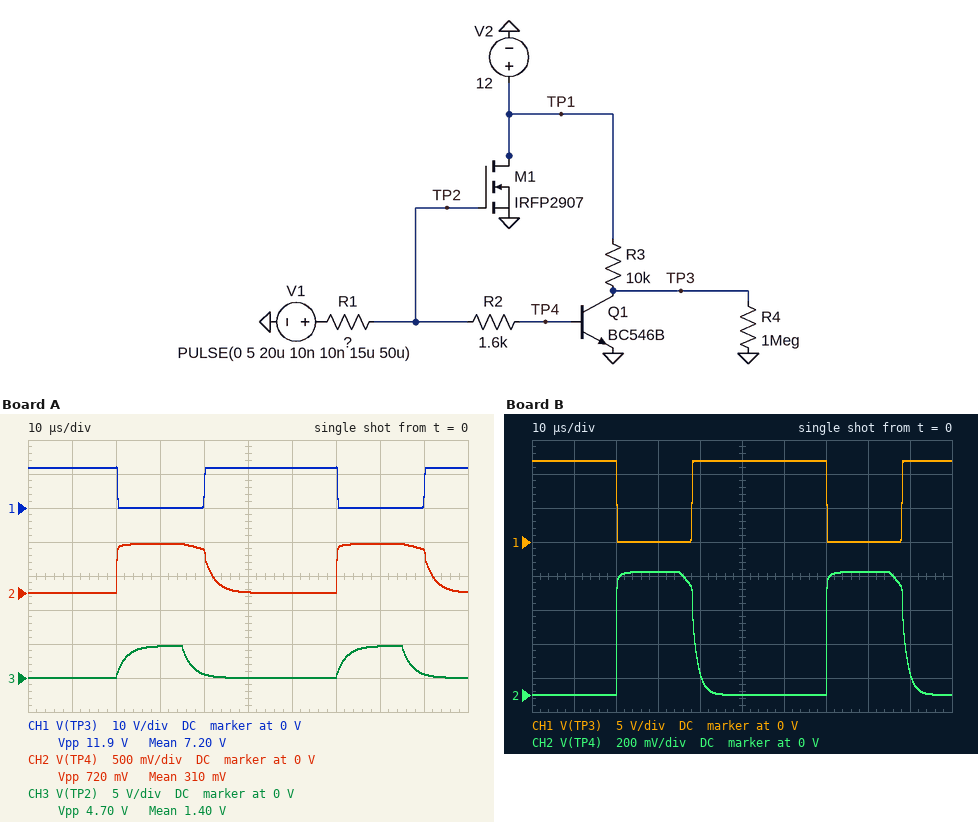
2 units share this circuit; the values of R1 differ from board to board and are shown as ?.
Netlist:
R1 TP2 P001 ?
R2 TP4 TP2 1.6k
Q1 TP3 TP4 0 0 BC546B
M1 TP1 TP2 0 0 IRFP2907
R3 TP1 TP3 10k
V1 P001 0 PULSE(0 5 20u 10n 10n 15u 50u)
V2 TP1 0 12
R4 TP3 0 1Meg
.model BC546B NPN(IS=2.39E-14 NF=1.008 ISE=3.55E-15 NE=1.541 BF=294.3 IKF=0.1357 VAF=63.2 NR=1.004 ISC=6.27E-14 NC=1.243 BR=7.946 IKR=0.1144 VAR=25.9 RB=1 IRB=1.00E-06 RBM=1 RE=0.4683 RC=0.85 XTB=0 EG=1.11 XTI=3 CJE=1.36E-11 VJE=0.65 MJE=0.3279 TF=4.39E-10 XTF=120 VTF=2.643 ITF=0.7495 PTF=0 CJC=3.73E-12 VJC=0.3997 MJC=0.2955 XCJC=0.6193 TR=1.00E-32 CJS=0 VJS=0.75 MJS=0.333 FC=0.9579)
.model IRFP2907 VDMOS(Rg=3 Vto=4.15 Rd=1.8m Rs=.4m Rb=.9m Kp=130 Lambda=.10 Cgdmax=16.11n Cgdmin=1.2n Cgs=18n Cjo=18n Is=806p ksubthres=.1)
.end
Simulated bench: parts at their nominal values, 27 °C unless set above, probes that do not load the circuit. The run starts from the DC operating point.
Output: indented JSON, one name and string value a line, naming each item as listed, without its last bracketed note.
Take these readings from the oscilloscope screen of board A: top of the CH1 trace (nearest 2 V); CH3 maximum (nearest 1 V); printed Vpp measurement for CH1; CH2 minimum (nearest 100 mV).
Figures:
{
  "top of the CH1 trace": "12 V",
  "CH3 maximum": "5 V",
  "printed Vpp measurement for CH1": "11.9 V",
  "CH2 minimum": "0 V"
}
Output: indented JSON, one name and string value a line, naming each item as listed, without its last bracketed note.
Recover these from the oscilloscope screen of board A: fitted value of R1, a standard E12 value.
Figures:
{
  "fitted value of R1, a standard E12 value": "120 Ω"
}
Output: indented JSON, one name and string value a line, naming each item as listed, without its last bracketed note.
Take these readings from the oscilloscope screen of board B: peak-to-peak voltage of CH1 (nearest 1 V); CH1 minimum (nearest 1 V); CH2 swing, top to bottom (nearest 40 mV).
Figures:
{
  "peak-to-peak voltage of CH1": "12 V",
  "CH1 minimum": "0 V",
  "CH2 swing, top to bottom": "720 mV"
}
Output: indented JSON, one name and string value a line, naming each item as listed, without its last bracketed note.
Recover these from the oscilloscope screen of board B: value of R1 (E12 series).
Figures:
{
  "value of R1": "68 Ω"
}
